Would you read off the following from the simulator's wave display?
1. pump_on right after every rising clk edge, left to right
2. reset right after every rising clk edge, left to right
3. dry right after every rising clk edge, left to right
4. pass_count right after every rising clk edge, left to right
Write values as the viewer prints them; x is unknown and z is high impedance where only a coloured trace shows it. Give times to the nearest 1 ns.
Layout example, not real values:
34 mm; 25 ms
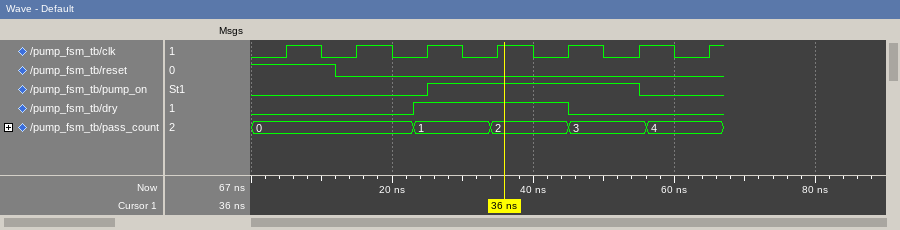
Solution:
0 0 1 1 1 0 0; 1 0 0 0 0 0 0; 0 0 1 1 0 0 0; 0, 0, 1, 2, 3, 3, 4
